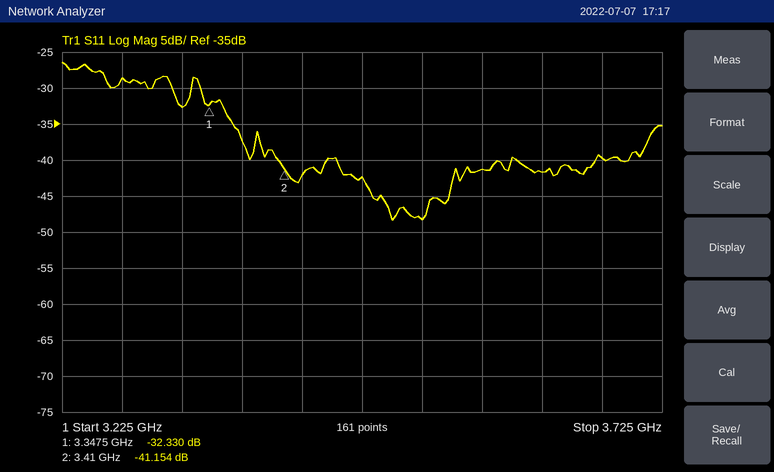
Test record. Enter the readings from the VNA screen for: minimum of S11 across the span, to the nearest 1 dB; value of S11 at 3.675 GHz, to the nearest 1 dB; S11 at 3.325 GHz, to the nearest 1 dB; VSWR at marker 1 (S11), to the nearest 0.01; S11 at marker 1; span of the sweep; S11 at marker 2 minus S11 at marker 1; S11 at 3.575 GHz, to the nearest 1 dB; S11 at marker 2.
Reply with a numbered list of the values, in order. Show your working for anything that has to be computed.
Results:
1. -48 dB
2. -40 dB
3. -33 dB
4. (1 + 0.0242)/(1 − 0.0242) ≈ 1.05
5. -32.330 dB
6. 500 MHz
7. -41.154 − (-32.33) = -8.824 dB
8. -41 dB
9. -41.154 dB
